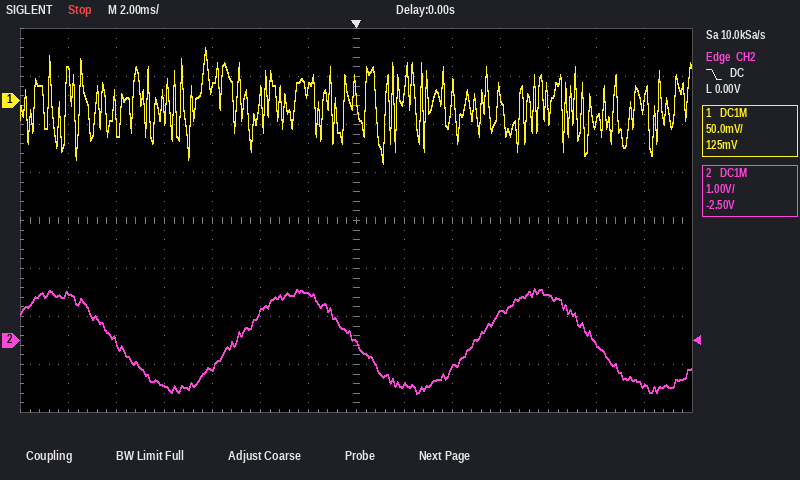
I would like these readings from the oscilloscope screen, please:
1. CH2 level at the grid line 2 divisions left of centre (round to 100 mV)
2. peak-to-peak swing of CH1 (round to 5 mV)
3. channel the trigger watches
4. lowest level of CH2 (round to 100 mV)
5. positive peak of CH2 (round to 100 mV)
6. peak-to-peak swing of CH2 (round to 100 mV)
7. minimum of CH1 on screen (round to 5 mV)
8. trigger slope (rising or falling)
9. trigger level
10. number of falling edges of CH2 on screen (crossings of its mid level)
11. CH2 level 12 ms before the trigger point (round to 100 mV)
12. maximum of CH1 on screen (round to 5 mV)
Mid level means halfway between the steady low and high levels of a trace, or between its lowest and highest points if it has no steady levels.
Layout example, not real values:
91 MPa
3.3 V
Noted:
600 mV
120 mV
CH2
-1.1 V
1.1 V
2.2 V
-65 mV
falling
0.00 V
3
1.0 V
55 mV
